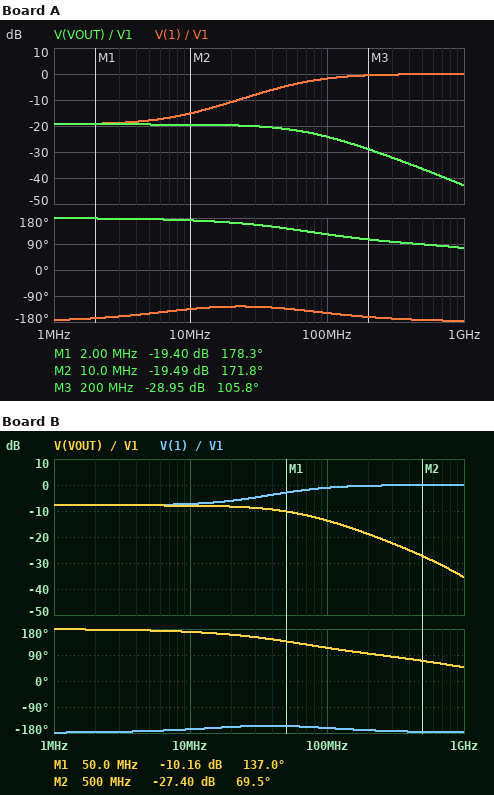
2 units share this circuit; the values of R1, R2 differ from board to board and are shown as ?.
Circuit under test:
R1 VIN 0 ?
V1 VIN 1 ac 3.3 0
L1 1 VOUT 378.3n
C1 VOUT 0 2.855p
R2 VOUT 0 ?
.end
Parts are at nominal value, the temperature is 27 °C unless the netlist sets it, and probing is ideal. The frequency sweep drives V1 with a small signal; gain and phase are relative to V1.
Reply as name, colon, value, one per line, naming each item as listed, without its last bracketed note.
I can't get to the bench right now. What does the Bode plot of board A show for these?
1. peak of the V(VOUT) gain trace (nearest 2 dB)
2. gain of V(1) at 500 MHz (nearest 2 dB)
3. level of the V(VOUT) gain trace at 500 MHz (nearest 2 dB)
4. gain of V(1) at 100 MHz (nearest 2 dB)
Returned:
peak of the V(VOUT) gain trace: -20 dB
gain of V(1) at 500 MHz: 0 dB
level of the V(VOUT) gain trace at 500 MHz: -36 dB
gain of V(1) at 100 MHz: -2 dB
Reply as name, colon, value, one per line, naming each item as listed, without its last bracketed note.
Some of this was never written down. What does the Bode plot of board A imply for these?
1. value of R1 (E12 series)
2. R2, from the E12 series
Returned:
value of R1: 150 Ω
R2, from the E12 series: 18 Ω
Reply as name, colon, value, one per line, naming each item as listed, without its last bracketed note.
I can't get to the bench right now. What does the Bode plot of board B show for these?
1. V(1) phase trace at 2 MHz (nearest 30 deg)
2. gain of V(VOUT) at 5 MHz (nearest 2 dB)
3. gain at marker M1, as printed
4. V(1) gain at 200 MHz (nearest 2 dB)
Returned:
V(1) phase trace at 2 MHz: -180 deg
gain of V(VOUT) at 5 MHz: -8 dB
gain at marker M1, as printed: -10.16 dB
V(1) gain at 200 MHz: 0 dB
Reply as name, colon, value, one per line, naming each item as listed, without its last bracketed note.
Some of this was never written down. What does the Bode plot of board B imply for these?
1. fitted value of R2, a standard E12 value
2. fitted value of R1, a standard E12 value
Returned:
fitted value of R2, a standard E12 value: 56 Ω
fitted value of R1, a standard E12 value: 82 Ω
